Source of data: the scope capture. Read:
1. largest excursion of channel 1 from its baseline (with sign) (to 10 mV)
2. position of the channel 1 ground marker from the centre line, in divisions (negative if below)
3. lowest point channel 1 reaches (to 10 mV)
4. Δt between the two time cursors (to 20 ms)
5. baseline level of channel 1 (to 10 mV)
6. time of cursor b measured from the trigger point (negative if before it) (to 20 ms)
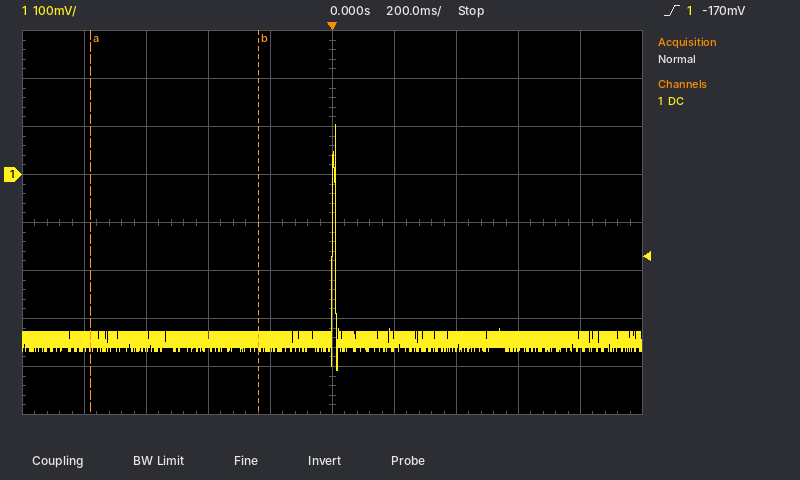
+450 mV
+1.0 div
-410 mV
540 ms
-340 mV
-240 ms
